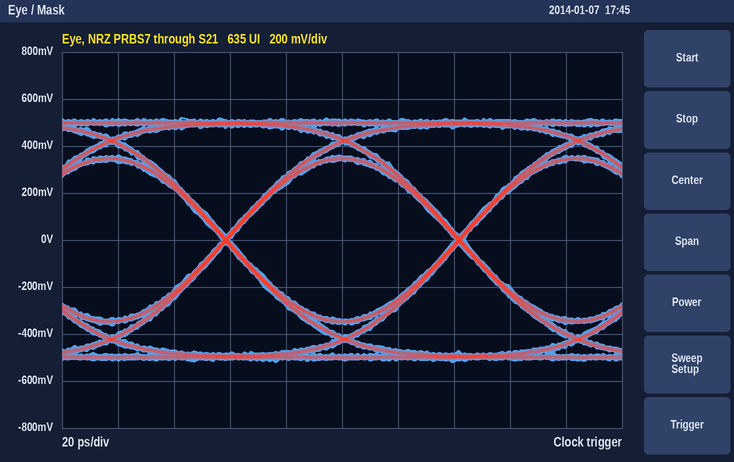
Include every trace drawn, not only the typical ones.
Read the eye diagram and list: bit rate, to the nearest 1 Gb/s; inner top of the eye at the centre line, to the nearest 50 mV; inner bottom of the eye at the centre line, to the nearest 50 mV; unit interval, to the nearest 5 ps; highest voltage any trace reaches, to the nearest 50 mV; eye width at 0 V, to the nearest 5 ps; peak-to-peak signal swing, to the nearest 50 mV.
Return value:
12 Gb/s
350 mV
-350 mV
85 ps
500 mV
80 ps
1.05 V
